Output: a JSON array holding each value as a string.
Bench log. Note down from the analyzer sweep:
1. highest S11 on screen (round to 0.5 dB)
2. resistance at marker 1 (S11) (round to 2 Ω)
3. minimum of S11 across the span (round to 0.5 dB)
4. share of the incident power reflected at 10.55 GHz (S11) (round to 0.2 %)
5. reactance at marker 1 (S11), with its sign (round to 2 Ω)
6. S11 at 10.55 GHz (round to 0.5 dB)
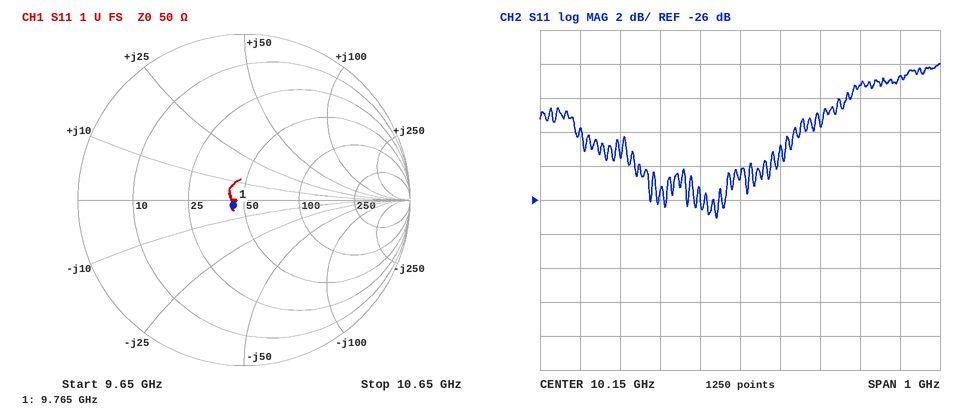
["-18.0 dB", "44 Ω", "-27.0 dB", "1.4 %", "-2 Ω", "-18.5 dB"]
